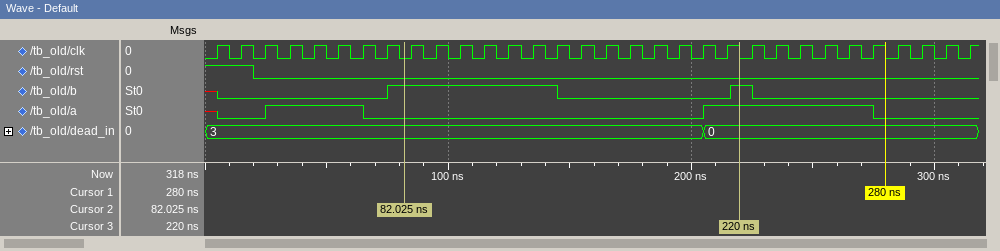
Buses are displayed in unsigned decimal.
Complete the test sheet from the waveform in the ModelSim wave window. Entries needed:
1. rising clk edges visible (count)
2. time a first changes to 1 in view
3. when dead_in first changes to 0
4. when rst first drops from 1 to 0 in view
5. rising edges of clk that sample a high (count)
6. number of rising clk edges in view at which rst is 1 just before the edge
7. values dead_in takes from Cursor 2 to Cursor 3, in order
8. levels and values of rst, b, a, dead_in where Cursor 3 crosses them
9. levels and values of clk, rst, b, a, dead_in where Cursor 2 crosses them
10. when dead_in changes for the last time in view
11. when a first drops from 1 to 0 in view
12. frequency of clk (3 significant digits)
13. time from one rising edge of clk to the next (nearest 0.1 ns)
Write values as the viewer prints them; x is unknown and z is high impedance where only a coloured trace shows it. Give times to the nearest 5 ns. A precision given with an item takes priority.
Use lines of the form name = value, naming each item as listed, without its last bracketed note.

rising clk edges visible = 32
time a first changes to 1 in view = 25 ns
when dead_in first changes to 0 = 205 ns
when rst first drops from 1 to 0 in view = 20 ns
rising edges of clk that sample a high = 11
number of rising clk edges in view at which rst is 1 just before the edge = 2
values dead_in takes from Cursor 2 to Cursor 3, in order = 3, 0
levels and values of rst, b, a, dead_in where Cursor 3 crosses them = rst=0, b=1, a=1, dead_in=0
levels and values of clk, rst, b, a, dead_in where Cursor 2 crosses them = clk=0, rst=0, b=1, a=0, dead_in=3
when dead_in changes for the last time in view = 205 ns
when a first drops from 1 to 0 in view = 65 ns
frequency of clk = 100 MHz
time from one rising edge of clk to the next = 10 ns
